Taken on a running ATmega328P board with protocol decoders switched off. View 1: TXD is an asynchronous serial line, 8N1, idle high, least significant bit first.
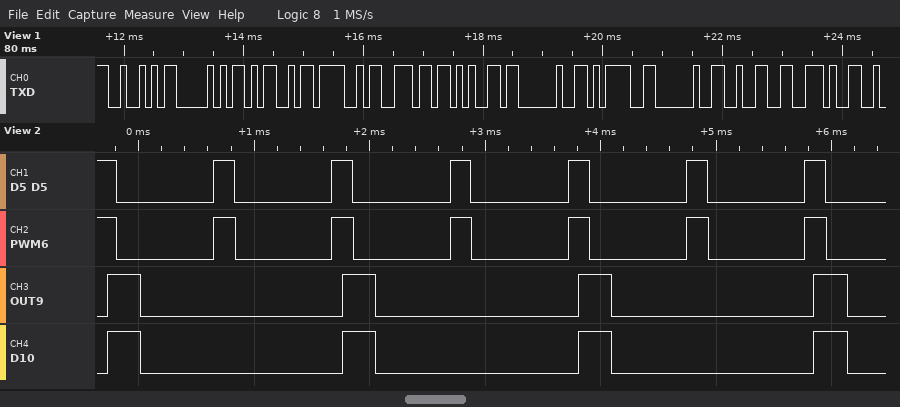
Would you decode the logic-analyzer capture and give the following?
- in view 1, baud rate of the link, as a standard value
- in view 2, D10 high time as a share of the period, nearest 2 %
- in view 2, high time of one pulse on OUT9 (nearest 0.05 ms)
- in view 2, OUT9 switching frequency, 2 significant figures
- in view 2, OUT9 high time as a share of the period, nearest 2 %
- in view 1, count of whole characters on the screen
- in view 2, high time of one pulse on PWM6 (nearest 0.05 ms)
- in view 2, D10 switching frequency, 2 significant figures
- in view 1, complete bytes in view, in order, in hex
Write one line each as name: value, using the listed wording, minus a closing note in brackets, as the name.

in view 1, baud rate of the link, as a standard value: 9600 baud
in view 2, D10 high time as a share of the period, nearest 2 %: 14 %
in view 2, high time of one pulse on OUT9: 0.30 ms
in view 2, OUT9 switching frequency, 2 significant figures: 490 Hz
in view 2, OUT9 high time as a share of the period, nearest 2 %: 14 %
in view 1, count of whole characters on the screen: 11
in view 2, high time of one pulse on PWM6: 0.20 ms
in view 2, D10 switching frequency, 2 significant figures: 490 Hz
in view 1, complete bytes in view, in order, in hex: 52 50 4D 4F 6E 65 20 3D 20 32 2E
